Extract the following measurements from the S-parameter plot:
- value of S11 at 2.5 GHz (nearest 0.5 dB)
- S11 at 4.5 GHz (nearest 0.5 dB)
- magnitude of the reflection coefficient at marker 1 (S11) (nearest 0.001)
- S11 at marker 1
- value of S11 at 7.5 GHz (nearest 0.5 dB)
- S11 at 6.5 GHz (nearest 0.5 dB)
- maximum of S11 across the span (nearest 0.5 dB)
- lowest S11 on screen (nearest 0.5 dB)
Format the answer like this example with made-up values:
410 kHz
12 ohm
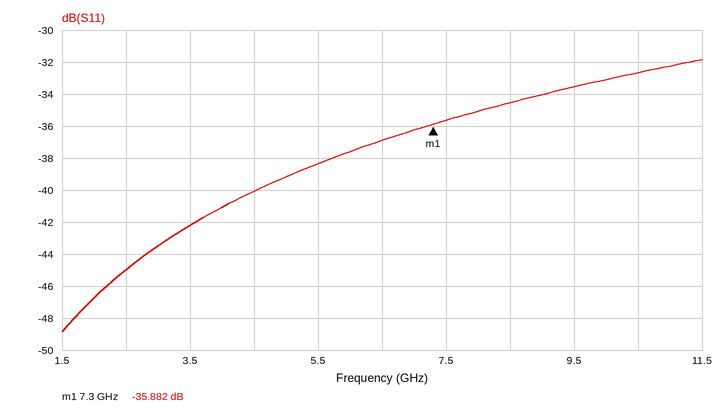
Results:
-45.0 dB
-40.0 dB
0.016
-35.882 dB
-35.5 dB
-37.0 dB
-32.0 dB
-49.0 dB
